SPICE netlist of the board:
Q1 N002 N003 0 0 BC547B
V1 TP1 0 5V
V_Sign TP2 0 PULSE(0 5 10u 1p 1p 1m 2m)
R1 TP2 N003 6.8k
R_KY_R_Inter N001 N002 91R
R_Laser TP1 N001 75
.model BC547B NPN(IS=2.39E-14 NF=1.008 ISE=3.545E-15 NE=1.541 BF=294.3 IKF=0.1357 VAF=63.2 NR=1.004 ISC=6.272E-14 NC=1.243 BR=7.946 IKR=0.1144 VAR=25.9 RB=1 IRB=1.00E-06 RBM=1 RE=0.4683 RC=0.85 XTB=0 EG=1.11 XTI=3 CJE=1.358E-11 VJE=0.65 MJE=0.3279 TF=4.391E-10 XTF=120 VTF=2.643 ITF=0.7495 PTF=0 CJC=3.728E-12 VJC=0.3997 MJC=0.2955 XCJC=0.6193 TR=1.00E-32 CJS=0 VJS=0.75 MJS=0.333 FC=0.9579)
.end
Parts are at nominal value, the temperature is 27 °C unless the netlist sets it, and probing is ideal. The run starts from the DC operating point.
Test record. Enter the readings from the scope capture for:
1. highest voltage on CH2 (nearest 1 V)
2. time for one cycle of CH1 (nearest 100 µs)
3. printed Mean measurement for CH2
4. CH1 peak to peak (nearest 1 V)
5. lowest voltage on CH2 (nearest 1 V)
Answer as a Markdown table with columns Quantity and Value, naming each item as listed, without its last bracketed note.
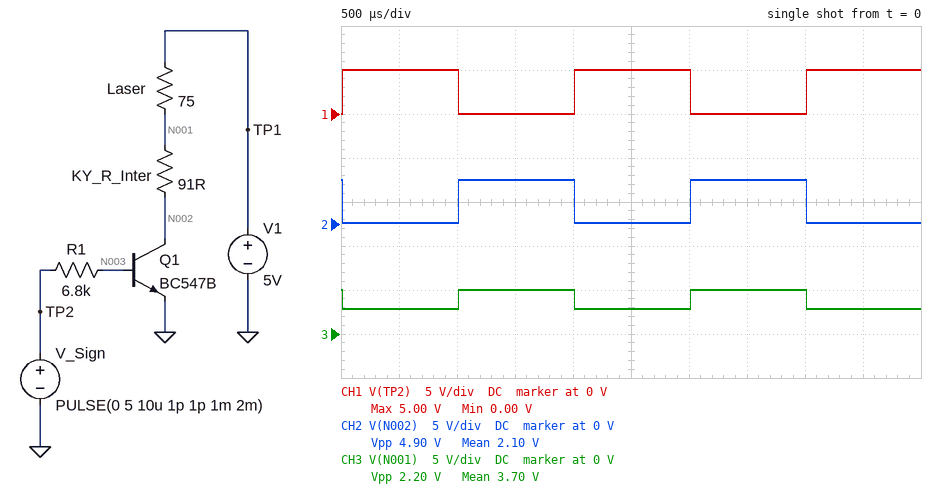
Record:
| Quantity | Value |
|---|---|
| highest voltage on CH2 | 5 V |
| time for one cycle of CH1 | 2.0 ms |
| printed Mean measurement for CH2 | 2.10 V |
| CH1 peak to peak | 5 V |
| lowest voltage on CH2 | 0 V |
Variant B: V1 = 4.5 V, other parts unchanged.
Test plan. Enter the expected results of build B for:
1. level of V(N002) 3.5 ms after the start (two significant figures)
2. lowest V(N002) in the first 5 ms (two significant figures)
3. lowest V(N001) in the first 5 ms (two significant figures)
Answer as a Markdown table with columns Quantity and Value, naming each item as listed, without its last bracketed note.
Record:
| Quantity | Value |
|---|---|
| level of V(N002) 3.5 ms after the start | 4.5 V |
| lowest V(N002) in the first 5 ms | 100 mV |
| lowest V(N001) in the first 5 ms | 2.5 V |
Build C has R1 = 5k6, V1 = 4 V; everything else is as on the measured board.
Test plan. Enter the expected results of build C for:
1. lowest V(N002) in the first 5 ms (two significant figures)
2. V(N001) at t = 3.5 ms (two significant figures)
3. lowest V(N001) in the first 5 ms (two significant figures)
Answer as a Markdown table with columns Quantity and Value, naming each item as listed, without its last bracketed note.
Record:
| Quantity | Value |
|---|---|
| lowest V(N002) in the first 5 ms | 88 mV |
| V(N001) at t = 3.5 ms | 4.0 V |
| lowest V(N001) in the first 5 ms | 2.2 V |
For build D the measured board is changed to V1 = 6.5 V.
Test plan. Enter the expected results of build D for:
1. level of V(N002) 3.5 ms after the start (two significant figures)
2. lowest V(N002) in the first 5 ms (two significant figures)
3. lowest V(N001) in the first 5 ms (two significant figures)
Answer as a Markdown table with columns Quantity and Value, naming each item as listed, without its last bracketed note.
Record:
| Quantity | Value |
|---|---|
| level of V(N002) 3.5 ms after the start | 6.5 V |
| lowest V(N002) in the first 5 ms | 130 mV |
| lowest V(N001) in the first 5 ms | 3.6 V |
